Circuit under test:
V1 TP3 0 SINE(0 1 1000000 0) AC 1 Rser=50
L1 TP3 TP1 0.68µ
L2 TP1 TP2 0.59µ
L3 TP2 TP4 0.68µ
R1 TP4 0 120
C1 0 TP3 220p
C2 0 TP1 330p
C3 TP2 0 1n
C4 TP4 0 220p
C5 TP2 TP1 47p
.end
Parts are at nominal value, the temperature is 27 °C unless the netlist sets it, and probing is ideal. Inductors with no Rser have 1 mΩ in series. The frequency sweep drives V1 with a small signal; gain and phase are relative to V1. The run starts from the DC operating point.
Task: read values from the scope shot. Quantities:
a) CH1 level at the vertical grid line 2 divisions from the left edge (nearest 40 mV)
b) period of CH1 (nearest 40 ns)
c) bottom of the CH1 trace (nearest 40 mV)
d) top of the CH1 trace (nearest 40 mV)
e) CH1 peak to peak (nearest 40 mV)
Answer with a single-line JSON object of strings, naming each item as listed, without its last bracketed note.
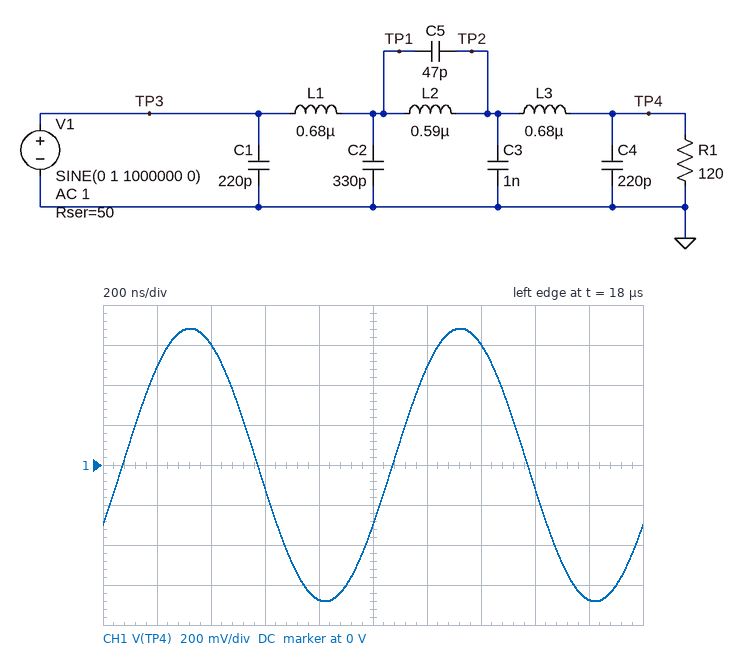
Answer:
{"CH1 level at the vertical grid line 2 divisions from the left edge": "600 mV", "period of CH1": "1.00 µs", "bottom of the CH1 trace": "-680 mV", "top of the CH1 trace": "680 mV", "CH1 peak to peak": "1.36 V"}
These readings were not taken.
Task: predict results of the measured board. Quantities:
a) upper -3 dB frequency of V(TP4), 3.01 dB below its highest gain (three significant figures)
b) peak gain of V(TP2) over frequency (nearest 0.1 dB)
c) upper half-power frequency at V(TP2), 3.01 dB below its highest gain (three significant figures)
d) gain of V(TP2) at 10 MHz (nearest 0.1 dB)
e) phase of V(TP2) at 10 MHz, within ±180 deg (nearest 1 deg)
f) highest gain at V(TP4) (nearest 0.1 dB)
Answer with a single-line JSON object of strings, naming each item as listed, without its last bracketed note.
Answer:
{"upper -3 dB frequency of V(TP4), 3.01 dB below its highest gain": "6.35 MHz", "peak gain of V(TP2) over frequency": "-3.0 dB", "upper half-power frequency at V(TP2), 3.01 dB below its highest gain": "3.89 MHz", "gain of V(TP2) at 10 MHz": "-12.2 dB", "phase of V(TP2) at 10 MHz, within ±180 deg": "-172 deg", "highest gain at V(TP4)": "-3.0 dB"}
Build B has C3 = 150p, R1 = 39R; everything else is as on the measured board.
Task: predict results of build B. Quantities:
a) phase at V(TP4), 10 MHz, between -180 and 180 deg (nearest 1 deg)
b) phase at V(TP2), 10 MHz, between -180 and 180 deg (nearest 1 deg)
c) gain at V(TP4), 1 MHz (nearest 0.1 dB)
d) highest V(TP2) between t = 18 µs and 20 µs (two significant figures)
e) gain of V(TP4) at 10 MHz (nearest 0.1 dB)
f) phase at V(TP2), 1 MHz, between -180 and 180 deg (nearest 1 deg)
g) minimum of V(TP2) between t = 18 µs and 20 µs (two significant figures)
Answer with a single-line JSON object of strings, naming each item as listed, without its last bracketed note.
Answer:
{"phase at V(TP4), 10 MHz, between -180 and 180 deg": "-161 deg", "phase at V(TP2), 10 MHz, between -180 and 180 deg": "-91 deg", "gain at V(TP4), 1 MHz": "-7.2 dB", "highest V(TP2) between t = 18 µs and 20 µs": "440 mV", "gain of V(TP4) at 10 MHz": "-8.2 dB", "phase at V(TP2), 1 MHz, between -180 and 180 deg": "-9 deg", "minimum of V(TP2) between t = 18 µs and 20 µs": "-440 mV"}
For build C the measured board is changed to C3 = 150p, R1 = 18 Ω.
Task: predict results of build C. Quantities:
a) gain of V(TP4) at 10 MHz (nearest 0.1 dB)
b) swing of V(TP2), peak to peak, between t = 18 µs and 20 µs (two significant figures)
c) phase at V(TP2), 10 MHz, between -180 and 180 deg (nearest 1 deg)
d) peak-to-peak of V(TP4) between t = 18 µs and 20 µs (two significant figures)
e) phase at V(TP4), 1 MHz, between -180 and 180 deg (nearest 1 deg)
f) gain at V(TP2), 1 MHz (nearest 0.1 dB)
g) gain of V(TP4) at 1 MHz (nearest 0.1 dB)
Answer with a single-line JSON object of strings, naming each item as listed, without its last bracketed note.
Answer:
{"gain of V(TP4) at 10 MHz": "-13.4 dB", "swing of V(TP2), peak to peak, between t = 18 µs and 20 µs": "540 mV", "phase at V(TP2), 10 MHz, between -180 and 180 deg": "-77 deg", "peak-to-peak of V(TP4) between t = 18 µs and 20 µs": "530 mV", "phase at V(TP4), 1 MHz, between -180 and 180 deg": "-15 deg", "gain at V(TP2), 1 MHz": "-11.3 dB", "gain of V(TP4) at 1 MHz": "-11.5 dB"}
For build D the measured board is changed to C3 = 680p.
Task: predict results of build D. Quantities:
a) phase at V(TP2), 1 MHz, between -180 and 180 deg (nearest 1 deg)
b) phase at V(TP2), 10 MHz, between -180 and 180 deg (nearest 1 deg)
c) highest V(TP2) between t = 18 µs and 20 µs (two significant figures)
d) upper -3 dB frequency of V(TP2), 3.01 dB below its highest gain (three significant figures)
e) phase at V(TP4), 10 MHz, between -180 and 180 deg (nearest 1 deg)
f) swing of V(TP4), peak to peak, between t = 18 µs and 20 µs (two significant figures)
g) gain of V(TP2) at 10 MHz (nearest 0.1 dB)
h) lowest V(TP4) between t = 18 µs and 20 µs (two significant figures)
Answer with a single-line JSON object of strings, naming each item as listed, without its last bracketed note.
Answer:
{"phase at V(TP2), 1 MHz, between -180 and 180 deg": "-20 deg", "phase at V(TP2), 10 MHz, between -180 and 180 deg": "-160 deg", "highest V(TP2) between t = 18 µs and 20 µs": "690 mV", "upper -3 dB frequency of V(TP2), 3.01 dB below its highest gain": "5.49 MHz", "phase at V(TP4), 10 MHz, between -180 and 180 deg": "159 deg", "swing of V(TP4), peak to peak, between t = 18 µs and 20 µs": "1.4 V", "gain of V(TP2) at 10 MHz": "-10.3 dB", "lowest V(TP4) between t = 18 µs and 20 µs": "-690 mV"}
